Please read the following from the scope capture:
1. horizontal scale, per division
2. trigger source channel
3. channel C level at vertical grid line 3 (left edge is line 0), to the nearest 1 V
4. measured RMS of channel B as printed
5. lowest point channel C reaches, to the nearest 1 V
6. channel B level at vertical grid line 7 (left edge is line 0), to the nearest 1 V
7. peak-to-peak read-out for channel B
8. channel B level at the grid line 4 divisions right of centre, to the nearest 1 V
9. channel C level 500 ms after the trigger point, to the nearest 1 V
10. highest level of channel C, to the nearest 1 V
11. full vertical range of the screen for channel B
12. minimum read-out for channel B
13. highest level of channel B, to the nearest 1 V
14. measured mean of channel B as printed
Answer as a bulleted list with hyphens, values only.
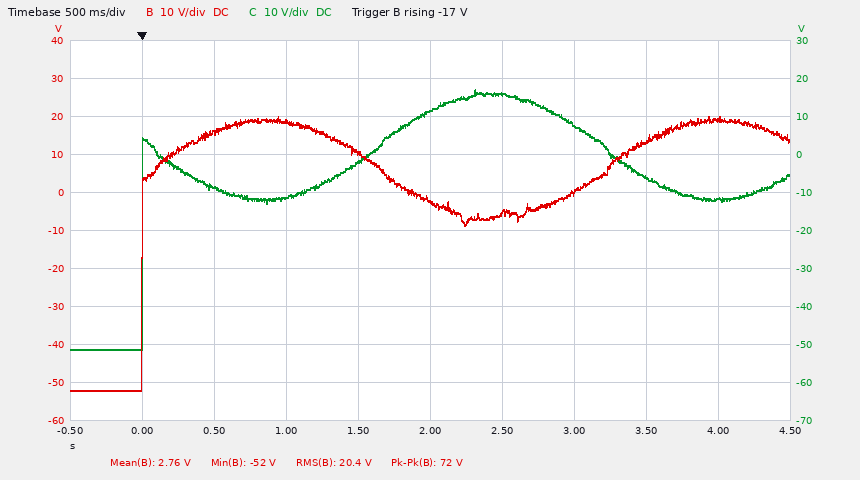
- 500 ms
- channel B
- -11 V
- 20.4 V
- -51 V
- 0 V
- 72 V
- 19 V
- -9 V
- 17 V
- 100 V
- -52 V
- 20 V
- 2.76 V
